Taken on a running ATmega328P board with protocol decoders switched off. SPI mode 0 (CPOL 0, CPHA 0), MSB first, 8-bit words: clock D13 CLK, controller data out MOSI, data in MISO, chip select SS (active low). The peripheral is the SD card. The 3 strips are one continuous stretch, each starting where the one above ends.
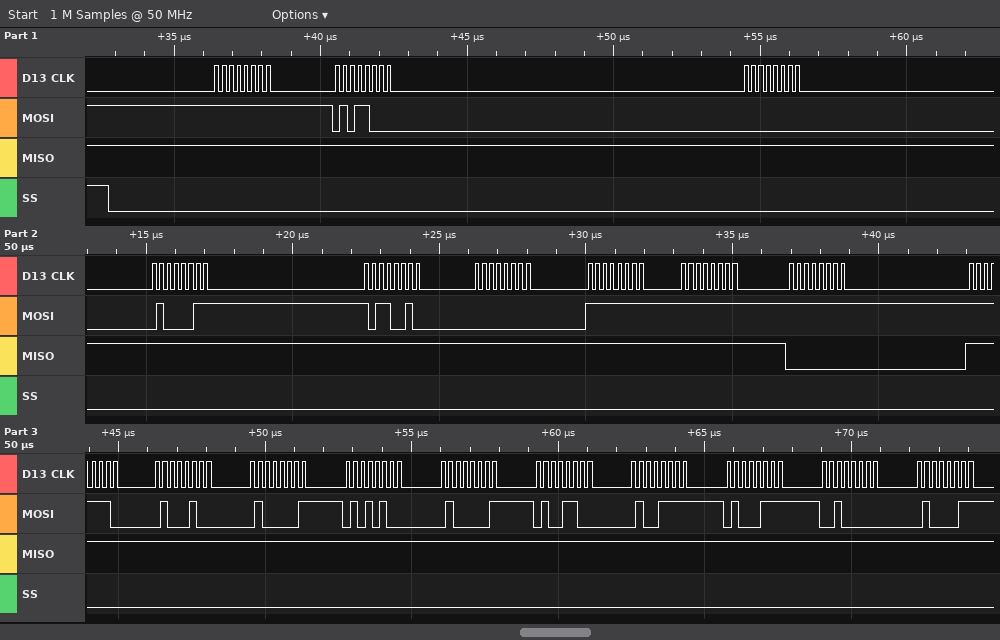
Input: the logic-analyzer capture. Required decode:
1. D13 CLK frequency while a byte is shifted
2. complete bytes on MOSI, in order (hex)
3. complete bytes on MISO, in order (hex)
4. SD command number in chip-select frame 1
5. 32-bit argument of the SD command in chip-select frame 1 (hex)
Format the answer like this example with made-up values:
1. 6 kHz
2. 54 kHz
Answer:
1. 4 MHz
2. 0xFF 0x58 0x00 0x43 0xB2 0x00 0xFF 0xFF 0xFF 0xFE 0x44 0x41 0x54 0x41 0x4C 0x4F 0x47 0x20 0x43
3. 0xFF 0xFF 0xFF 0xFF 0xFF 0xFF 0xFF 0xFF 0x00 0xFF 0xFF 0xFF 0xFF 0xFF 0xFF 0xFF 0xFF 0xFF 0xFF
4. CMD24
5. 0x0043B200
